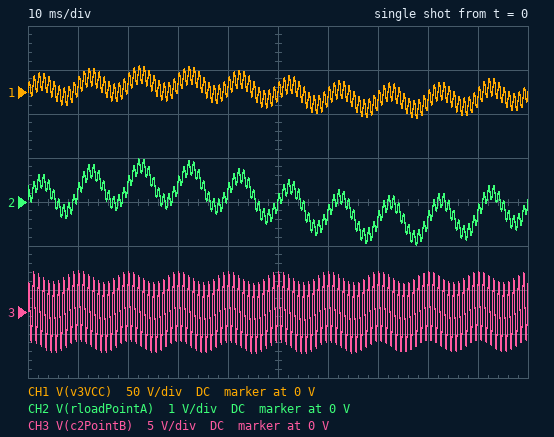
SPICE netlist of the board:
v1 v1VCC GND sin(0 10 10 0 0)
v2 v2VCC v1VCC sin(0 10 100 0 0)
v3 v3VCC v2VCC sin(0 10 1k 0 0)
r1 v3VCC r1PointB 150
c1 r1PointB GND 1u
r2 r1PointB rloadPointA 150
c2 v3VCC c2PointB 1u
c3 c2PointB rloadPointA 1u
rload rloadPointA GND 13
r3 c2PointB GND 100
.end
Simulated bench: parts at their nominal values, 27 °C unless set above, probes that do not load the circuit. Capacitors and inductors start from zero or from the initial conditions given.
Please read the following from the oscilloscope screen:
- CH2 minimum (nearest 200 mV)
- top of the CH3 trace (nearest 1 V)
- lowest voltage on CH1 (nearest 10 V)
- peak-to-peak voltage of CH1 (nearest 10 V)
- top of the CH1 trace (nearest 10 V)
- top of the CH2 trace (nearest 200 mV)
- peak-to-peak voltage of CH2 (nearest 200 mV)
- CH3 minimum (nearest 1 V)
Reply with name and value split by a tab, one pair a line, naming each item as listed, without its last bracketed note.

CH2 minimum	-1.0 V
top of the CH3 trace	5 V
lowest voltage on CH1	-30 V
peak-to-peak voltage of CH1	60 V
top of the CH1 trace	30 V
top of the CH2 trace	1.0 V
peak-to-peak voltage of CH2	2.0 V
CH3 minimum	-5 V
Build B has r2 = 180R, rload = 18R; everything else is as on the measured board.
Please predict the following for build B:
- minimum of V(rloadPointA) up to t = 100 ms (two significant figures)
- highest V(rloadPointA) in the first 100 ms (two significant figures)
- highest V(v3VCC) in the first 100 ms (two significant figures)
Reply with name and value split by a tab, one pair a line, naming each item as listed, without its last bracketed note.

minimum of V(rloadPointA) up to t = 100 ms	-1.2 V
highest V(rloadPointA) in the first 100 ms	1.2 V
highest V(v3VCC) in the first 100 ms	30 V
